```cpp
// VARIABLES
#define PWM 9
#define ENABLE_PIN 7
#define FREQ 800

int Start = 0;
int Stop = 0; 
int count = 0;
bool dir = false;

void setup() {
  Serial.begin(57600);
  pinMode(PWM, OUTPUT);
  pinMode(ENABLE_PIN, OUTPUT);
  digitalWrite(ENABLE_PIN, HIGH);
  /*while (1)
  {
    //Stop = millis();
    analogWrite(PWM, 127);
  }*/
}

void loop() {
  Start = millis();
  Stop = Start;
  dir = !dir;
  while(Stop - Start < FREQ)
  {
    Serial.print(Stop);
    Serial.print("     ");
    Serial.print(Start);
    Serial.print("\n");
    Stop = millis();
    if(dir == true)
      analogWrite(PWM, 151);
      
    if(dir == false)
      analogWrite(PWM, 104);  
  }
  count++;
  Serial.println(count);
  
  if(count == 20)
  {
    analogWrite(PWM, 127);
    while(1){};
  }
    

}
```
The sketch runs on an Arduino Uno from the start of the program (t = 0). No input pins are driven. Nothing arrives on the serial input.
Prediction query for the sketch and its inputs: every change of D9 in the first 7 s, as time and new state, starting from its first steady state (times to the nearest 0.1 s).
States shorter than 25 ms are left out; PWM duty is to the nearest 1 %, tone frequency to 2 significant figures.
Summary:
0 s PWM 59 %; 0.8 s PWM 41 %; 1.6 s PWM 59 %; 2.4 s PWM 41 %; 3.2 s PWM 59 %; 4 s PWM 41 %; 4.8 s PWM 59 %; 5.6 s PWM 41 %; 6.4 s PWM 59 %
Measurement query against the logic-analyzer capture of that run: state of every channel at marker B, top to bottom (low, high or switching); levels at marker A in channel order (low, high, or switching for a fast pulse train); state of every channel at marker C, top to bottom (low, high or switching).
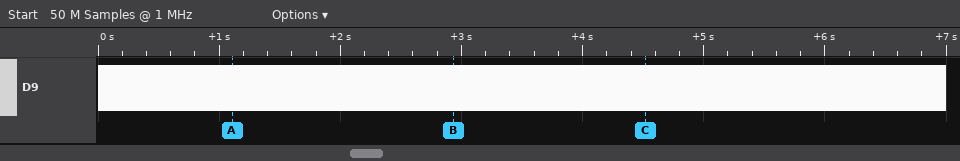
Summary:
D9 switching
D9 switching
D9 switching
